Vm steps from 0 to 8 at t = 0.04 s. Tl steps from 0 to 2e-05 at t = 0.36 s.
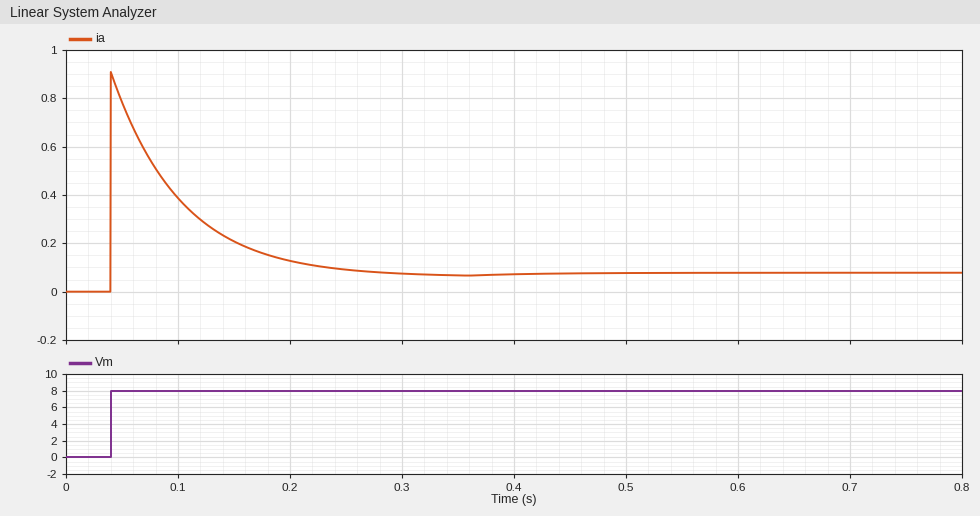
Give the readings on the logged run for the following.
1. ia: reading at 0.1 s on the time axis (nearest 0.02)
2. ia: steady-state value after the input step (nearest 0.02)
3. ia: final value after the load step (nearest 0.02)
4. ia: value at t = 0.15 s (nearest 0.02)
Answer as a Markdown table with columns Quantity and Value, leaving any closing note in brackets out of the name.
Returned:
| Quantity | Value |
|---|---|
| ia: reading at 0.1 s on the time axis | 0.38 |
| ia: steady-state value after the input step | 0.06 |
| ia: final value after the load step | 0.08 |
| ia: value at t = 0.15 s | 0.20 |
